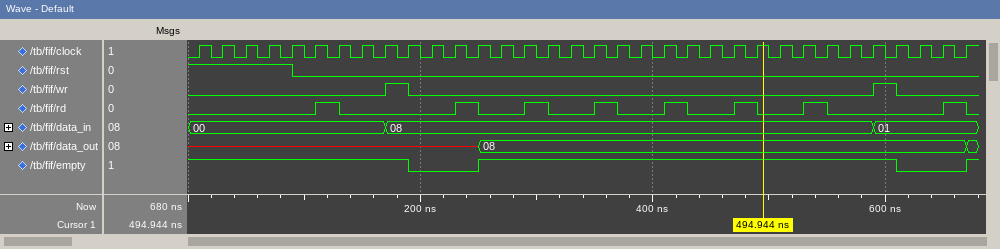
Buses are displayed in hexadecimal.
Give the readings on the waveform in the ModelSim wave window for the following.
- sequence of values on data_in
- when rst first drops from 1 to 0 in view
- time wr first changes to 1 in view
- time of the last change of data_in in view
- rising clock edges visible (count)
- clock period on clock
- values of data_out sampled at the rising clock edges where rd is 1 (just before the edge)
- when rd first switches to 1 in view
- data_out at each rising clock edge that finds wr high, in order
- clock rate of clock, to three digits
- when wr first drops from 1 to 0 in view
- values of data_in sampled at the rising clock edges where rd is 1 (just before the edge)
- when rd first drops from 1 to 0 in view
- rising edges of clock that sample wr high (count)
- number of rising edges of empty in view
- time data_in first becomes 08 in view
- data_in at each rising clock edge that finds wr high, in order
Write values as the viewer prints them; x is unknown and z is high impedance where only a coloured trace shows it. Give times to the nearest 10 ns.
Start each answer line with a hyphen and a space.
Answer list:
- 00, 08, 01
- 90 ns
- 170 ns
- 590 ns
- 34
- 20 ns
- x, x, 08, 08, 08, 08, 08, 08
- 110 ns
- x, 08
- 50.0 MHz
- 190 ns
- 00, 08, 08, 08, 08, 08, 08, 01
- 130 ns
- 2
- 2
- 170 ns
- 08, 01
